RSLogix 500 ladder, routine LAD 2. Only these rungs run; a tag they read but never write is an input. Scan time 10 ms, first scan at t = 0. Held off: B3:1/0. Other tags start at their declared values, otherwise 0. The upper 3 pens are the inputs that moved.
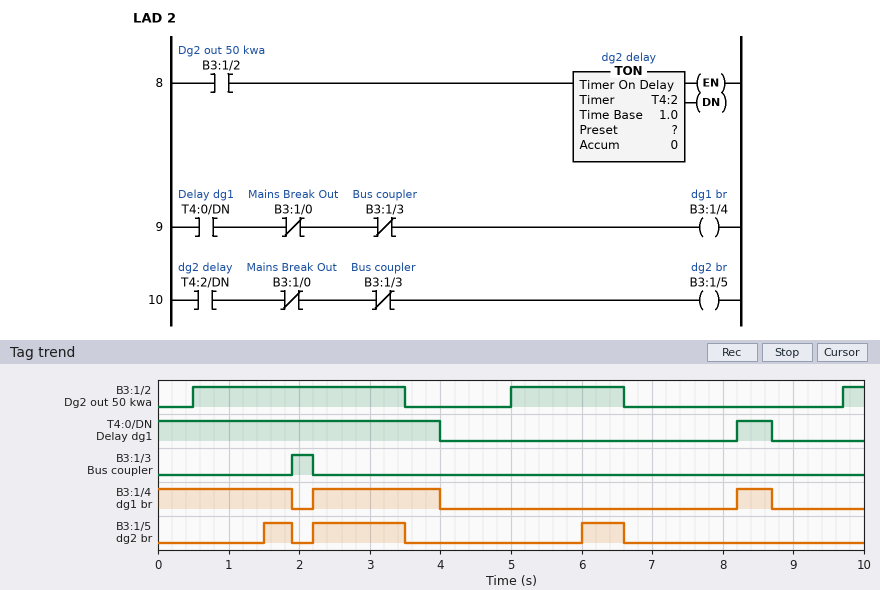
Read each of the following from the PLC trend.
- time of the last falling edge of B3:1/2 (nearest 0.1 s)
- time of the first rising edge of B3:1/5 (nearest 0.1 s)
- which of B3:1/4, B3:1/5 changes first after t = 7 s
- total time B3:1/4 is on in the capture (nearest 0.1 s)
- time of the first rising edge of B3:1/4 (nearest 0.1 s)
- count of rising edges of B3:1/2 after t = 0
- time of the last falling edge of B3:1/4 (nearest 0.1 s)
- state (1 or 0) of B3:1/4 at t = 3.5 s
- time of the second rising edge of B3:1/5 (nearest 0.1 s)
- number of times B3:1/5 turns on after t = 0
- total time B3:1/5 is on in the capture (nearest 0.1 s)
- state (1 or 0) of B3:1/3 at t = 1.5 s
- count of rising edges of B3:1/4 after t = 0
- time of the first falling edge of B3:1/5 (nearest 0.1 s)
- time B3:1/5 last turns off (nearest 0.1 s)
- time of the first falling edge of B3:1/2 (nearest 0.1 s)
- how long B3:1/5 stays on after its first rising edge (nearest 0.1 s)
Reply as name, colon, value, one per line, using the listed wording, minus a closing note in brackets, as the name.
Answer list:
time of the last falling edge of B3:1/2: 6.6 s
time of the first rising edge of B3:1/5: 1.5 s
which of B3:1/4, B3:1/5 changes first after t = 7 s: B3:1/4
total time B3:1/4 is on in the capture: 4.2 s
time of the first rising edge of B3:1/4: 2.2 s
count of rising edges of B3:1/2 after t = 0: 3
time of the last falling edge of B3:1/4: 8.7 s
state (1 or 0) of B3:1/4 at t = 3.5 s: 1
time of the second rising edge of B3:1/5: 2.2 s
number of times B3:1/5 turns on after t = 0: 3
total time B3:1/5 is on in the capture: 2.3 s
state (1 or 0) of B3:1/3 at t = 1.5 s: 0
count of rising edges of B3:1/4 after t = 0: 2
time of the first falling edge of B3:1/5: 1.9 s
time B3:1/5 last turns off: 6.6 s
time of the first falling edge of B3:1/2: 3.5 s
how long B3:1/5 stays on after its first rising edge: 0.4 s
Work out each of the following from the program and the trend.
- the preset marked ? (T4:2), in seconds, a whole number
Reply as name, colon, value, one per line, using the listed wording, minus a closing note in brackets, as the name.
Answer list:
the preset marked ? (T4:2), in seconds, a whole number: 1 s
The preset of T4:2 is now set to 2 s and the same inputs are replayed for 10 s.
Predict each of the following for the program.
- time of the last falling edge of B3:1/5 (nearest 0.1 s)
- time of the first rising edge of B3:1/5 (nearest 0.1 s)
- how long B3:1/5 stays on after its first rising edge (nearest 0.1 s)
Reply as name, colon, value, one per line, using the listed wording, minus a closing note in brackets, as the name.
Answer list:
time of the last falling edge of B3:1/5: 3.5 s
time of the first rising edge of B3:1/5: 2.5 s
how long B3:1/5 stays on after its first rising edge: 1.0 s
